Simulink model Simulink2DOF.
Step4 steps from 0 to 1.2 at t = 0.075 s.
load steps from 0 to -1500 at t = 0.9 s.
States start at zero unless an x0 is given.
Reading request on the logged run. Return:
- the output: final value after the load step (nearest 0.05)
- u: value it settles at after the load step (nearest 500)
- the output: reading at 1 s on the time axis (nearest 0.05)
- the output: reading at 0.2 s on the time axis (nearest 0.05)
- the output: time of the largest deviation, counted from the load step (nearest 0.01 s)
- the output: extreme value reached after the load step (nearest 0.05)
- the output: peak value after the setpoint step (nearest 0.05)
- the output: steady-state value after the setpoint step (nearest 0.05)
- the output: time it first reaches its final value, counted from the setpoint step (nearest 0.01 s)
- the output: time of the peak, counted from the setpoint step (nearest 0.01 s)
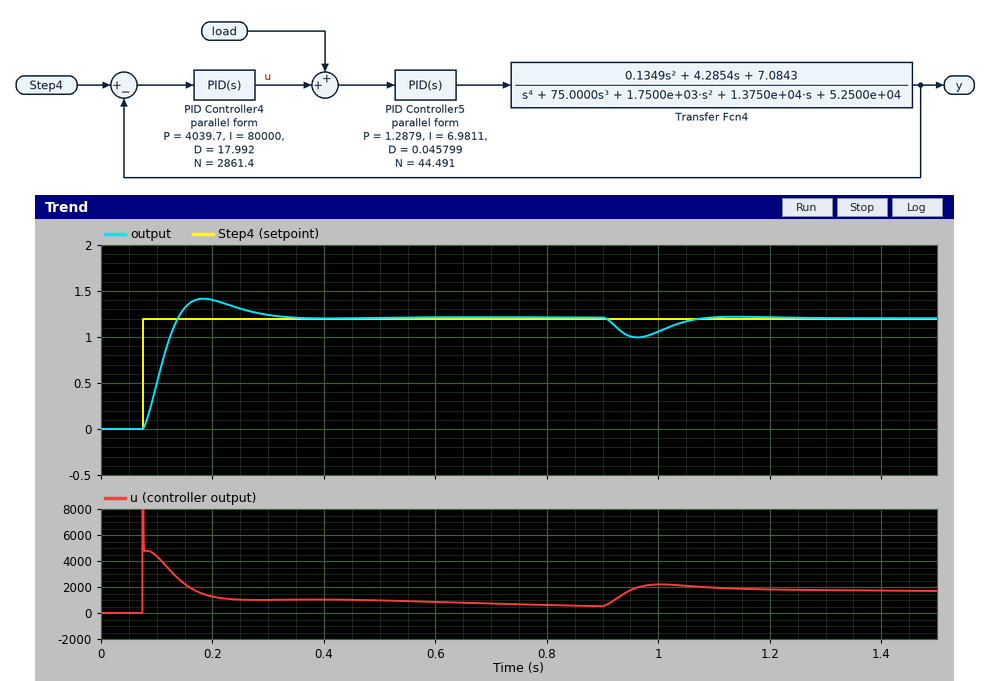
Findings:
1.20
1500
1.05
1.40
0.06 s
1.00
1.40
1.20
0.06 s
0.11 s
